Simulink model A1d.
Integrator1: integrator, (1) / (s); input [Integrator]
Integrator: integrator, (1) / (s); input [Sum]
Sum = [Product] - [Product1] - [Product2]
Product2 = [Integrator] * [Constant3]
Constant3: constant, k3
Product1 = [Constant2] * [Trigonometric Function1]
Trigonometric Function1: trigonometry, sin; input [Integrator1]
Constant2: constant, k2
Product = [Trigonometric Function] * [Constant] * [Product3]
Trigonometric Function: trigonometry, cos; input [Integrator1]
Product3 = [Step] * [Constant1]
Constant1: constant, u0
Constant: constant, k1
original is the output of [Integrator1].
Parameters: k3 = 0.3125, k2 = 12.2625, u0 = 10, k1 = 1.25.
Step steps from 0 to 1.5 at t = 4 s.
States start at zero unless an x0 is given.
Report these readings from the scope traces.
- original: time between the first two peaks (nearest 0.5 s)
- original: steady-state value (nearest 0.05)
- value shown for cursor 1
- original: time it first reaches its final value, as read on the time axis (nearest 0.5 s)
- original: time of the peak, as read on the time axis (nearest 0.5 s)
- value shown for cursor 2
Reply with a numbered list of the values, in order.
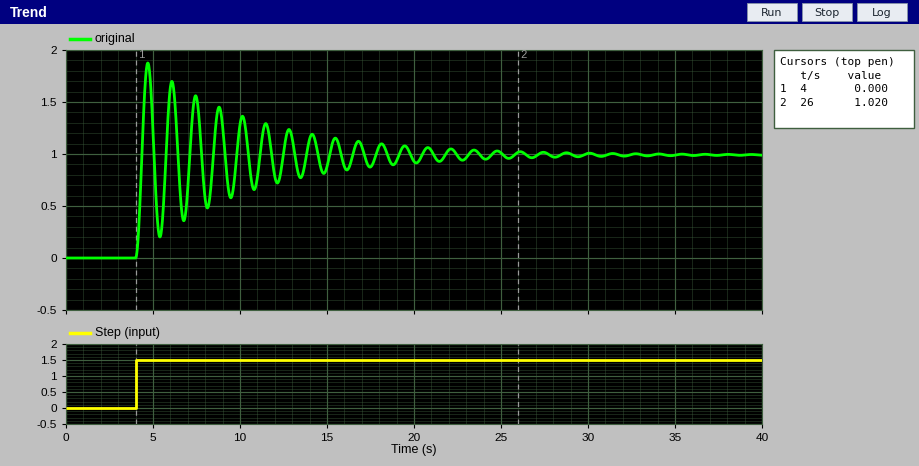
1. 1.5 s
2. 1.00
3. 0.000
4. 4.5 s
5. 4.5 s
6. 1.020
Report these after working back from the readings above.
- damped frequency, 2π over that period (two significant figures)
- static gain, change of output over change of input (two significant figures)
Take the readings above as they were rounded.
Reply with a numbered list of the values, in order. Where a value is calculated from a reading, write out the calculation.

1. 2π / 1.5 = 4.2 rad/s
2. (1 - 0) / (1.5 - 0) = 0.67
